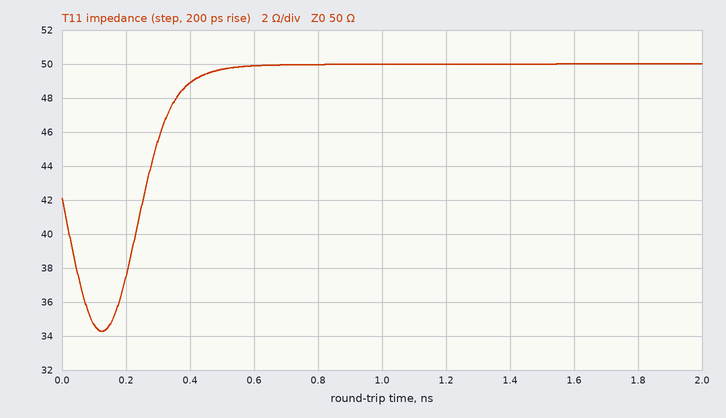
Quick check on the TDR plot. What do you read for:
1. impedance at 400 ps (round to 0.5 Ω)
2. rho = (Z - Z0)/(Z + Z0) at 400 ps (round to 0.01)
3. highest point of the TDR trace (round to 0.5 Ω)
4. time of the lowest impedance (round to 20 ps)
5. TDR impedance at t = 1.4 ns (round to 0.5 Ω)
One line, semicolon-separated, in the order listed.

49.0 Ω; -0.01; 50.0 Ω; 120 ps; 50.0 Ω
